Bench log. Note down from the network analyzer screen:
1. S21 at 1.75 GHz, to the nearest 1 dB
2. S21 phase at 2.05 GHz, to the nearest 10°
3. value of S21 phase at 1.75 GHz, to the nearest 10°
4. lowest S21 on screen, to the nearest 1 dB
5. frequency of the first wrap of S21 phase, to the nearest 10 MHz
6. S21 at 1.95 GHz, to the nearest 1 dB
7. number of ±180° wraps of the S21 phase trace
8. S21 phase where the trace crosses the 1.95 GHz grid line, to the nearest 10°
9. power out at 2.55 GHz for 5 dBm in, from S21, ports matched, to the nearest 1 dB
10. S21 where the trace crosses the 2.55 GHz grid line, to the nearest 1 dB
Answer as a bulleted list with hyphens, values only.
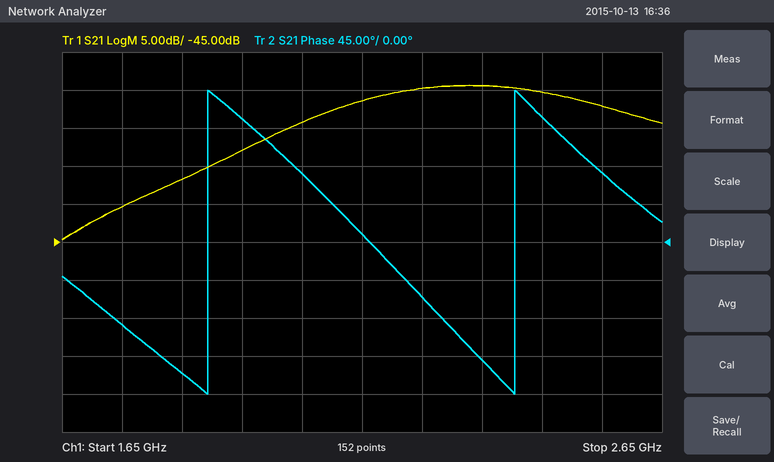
- -40 dB
- 80°
- -100°
- -45 dB
- 1.89 GHz
- -33 dB
- 2
- 150°
- -22 dBm
- -27 dB
